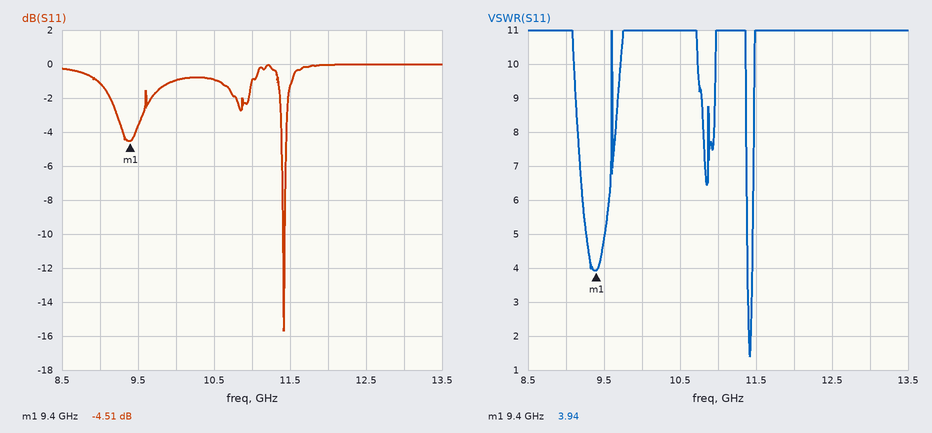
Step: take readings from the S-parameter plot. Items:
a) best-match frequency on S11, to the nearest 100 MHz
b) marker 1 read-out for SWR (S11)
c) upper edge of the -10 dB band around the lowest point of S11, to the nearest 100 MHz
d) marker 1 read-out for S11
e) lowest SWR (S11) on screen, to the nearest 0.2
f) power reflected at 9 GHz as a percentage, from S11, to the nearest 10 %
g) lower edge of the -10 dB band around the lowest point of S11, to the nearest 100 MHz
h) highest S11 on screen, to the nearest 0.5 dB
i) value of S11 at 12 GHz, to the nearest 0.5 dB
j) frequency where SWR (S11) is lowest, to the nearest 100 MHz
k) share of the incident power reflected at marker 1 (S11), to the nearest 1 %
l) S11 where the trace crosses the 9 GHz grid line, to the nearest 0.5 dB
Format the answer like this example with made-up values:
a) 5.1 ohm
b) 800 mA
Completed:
a) 11.4 GHz
b) 3.94
c) 11.4 GHz
d) -4.51 dB
e) 1.4
f) 80 %
g) 11.4 GHz
h) 0.0 dB
i) 0.0 dB
j) 11.4 GHz
k) 35 %
l) -1.0 dB
